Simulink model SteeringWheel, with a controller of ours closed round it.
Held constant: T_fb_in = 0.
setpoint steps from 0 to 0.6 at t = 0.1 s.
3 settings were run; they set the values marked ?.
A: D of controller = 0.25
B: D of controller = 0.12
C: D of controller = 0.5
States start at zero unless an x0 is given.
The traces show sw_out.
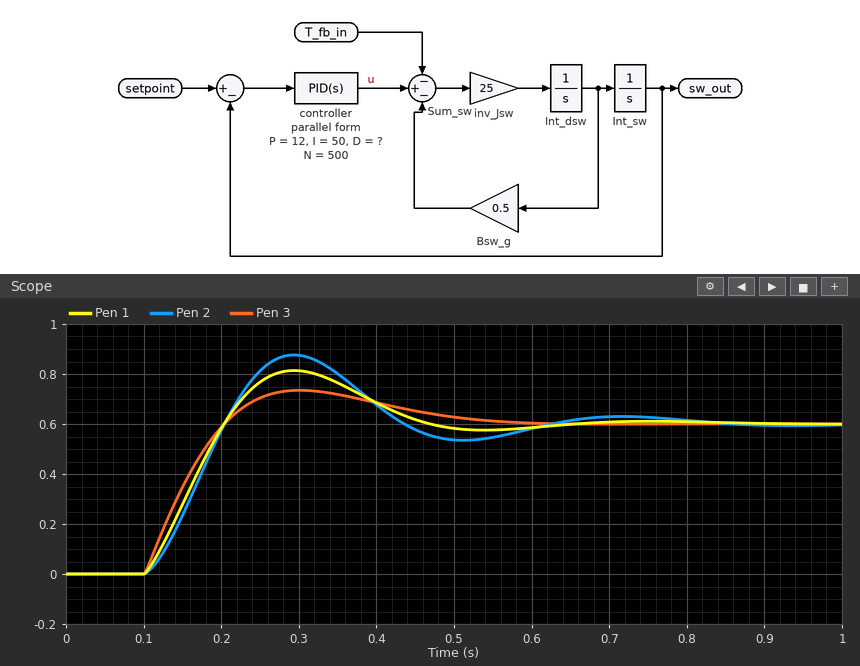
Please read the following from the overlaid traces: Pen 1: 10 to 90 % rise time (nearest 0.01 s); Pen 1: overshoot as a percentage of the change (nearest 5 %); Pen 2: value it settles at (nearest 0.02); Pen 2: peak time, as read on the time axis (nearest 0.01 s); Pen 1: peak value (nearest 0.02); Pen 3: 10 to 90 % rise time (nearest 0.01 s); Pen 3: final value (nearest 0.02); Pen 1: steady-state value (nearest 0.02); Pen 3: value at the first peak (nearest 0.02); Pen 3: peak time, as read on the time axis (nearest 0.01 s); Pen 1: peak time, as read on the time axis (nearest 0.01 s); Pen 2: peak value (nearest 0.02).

0.08 s
35 %
0.60
0.29 s
0.82
0.08 s
0.60
0.60
0.74
0.30 s
0.29 s
0.88
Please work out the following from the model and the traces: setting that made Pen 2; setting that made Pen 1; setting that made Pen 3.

B
A
C
